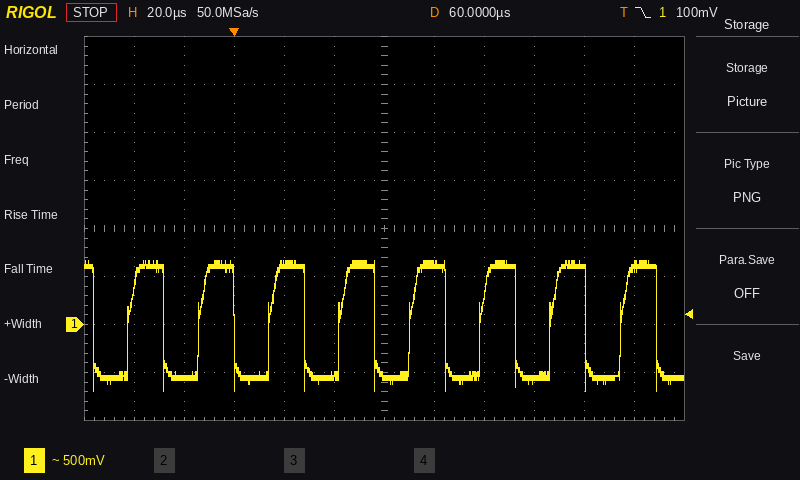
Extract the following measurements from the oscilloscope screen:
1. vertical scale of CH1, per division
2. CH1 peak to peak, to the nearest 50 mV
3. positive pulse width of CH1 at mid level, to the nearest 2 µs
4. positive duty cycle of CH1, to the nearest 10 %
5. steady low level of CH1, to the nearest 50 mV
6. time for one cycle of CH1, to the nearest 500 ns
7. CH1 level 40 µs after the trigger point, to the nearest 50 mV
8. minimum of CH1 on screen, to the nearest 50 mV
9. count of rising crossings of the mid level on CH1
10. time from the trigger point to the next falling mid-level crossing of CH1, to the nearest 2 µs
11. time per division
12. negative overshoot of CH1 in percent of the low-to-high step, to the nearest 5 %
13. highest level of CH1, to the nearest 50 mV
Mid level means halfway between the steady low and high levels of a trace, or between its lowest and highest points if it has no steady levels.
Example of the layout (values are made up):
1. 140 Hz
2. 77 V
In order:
1. 500 mV
2. 1.35 V
3. 14 µs
4. 50 %
5. -550 mV
6. 28.0 µs
7. -550 mV
8. -700 mV
9. 8
10. 28 µs
11. 20 µs
12. 10 %
13. 650 mV
